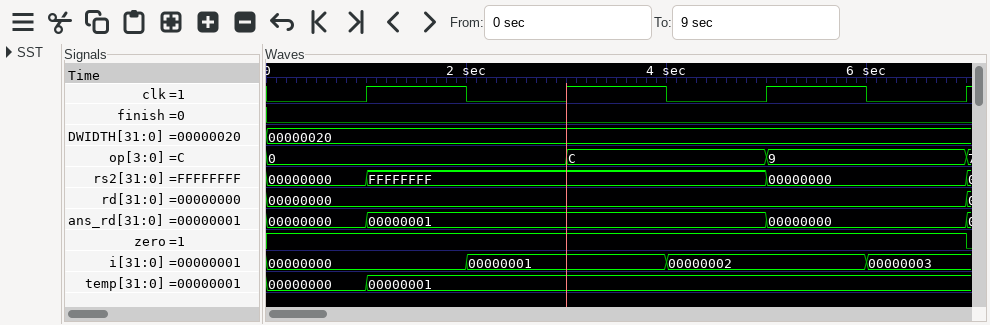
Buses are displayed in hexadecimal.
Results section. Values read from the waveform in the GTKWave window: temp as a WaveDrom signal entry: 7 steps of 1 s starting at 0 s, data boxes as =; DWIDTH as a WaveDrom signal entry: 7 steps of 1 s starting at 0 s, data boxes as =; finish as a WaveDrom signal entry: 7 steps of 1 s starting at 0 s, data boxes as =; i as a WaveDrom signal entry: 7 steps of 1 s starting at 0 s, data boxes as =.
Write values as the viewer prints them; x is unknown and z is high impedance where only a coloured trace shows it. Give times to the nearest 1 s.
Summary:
{name: 'temp', wave: '==.....', data: '00000000 00000001'}
{name: 'DWIDTH', wave: '=......', data: '00000020'}
{name: 'finish', wave: '0......'}
{name: 'i', wave: '=.=.=.=', data: '00000000 00000001 00000002 00000003'}
